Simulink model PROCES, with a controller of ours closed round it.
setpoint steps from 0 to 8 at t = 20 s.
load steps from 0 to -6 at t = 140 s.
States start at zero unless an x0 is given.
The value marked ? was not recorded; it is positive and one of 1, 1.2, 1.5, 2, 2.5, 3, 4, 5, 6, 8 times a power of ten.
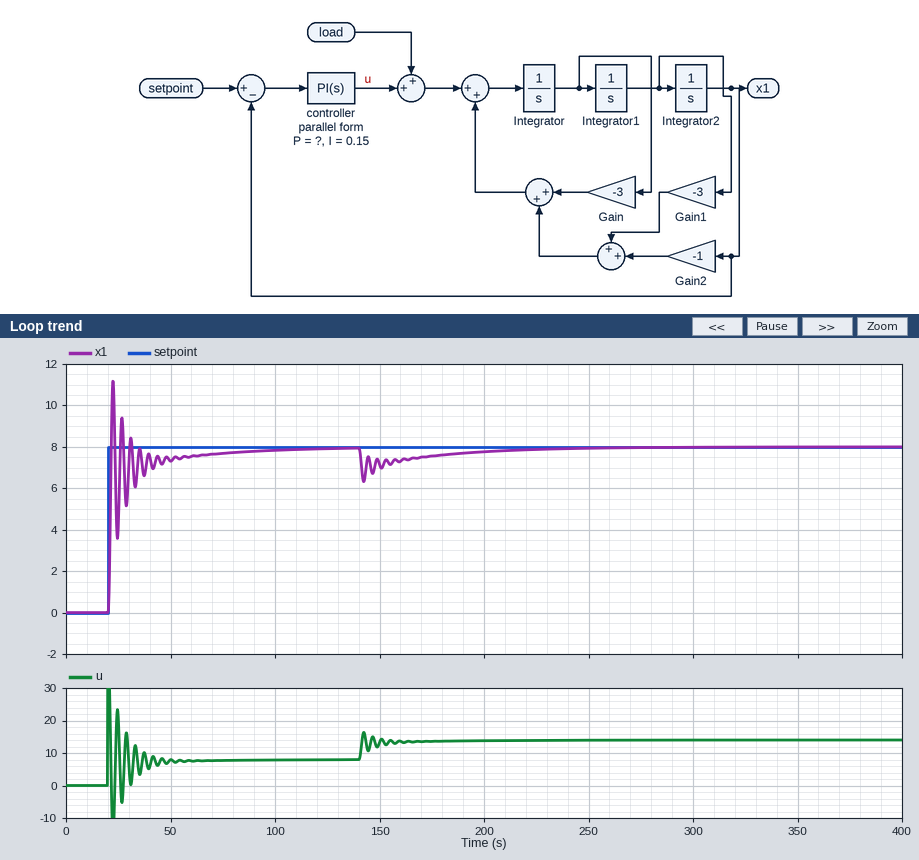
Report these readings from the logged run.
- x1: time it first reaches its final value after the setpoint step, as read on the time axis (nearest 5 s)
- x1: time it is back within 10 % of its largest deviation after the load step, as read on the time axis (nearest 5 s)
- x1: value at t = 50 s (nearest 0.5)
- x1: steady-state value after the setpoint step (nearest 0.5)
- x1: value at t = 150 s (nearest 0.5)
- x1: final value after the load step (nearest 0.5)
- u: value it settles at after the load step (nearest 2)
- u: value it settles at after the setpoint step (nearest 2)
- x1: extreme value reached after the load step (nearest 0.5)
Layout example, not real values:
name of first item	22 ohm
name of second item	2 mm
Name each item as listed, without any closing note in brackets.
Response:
x1: time it first reaches its final value after the setpoint step, as read on the time axis	20 s
x1: time it is back within 10 % of its largest deviation after the load step, as read on the time axis	215 s
x1: value at t = 50 s	7.5
x1: steady-state value after the setpoint step	8.0
x1: value at t = 150 s	7.0
x1: final value after the load step	8.0
u: value it settles at after the load step	14
u: value it settles at after the setpoint step	8
x1: extreme value reached after the load step	6.5
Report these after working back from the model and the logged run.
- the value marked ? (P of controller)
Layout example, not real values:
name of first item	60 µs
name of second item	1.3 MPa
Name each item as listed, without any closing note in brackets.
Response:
the value marked ?	5
